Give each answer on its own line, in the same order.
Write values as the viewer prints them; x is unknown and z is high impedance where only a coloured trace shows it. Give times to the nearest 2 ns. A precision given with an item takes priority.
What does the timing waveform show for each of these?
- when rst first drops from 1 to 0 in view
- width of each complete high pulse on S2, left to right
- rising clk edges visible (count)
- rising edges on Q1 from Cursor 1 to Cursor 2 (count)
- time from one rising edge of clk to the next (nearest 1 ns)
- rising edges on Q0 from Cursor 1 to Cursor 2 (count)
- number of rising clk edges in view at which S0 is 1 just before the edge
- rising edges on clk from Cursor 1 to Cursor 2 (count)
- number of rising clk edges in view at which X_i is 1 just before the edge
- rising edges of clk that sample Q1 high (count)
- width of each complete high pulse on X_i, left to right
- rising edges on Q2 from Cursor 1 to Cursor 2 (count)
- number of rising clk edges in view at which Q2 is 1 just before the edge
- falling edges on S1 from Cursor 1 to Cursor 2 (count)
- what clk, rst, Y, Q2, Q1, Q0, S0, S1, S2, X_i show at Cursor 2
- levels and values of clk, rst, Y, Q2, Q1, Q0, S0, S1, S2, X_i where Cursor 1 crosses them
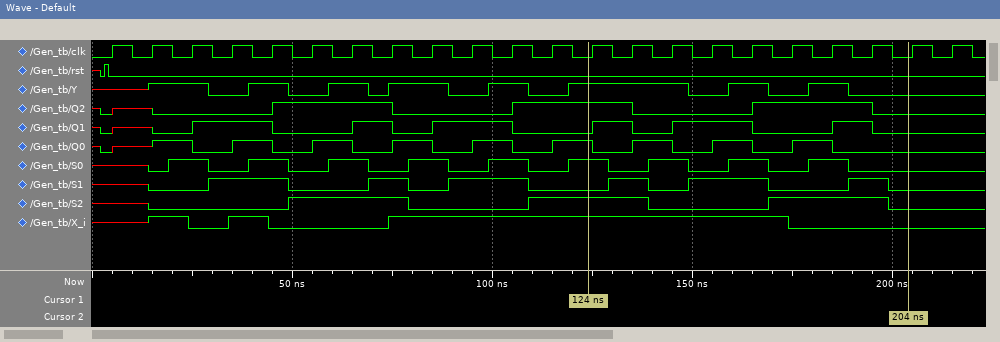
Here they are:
4 ns
30 ns, 30 ns, 30 ns
22
3
10 ns
3
9
8
12
9
10 ns, 100 ns
1
9
3
clk=0, rst=0, Y=0, Q2=0, Q1=0, Q0=0, S0=0, S1=0, S2=0, X_i=0
clk=0, rst=0, Y=1, Q2=1, Q1=0, Q0=1, S0=1, S1=0, S2=1, X_i=1
